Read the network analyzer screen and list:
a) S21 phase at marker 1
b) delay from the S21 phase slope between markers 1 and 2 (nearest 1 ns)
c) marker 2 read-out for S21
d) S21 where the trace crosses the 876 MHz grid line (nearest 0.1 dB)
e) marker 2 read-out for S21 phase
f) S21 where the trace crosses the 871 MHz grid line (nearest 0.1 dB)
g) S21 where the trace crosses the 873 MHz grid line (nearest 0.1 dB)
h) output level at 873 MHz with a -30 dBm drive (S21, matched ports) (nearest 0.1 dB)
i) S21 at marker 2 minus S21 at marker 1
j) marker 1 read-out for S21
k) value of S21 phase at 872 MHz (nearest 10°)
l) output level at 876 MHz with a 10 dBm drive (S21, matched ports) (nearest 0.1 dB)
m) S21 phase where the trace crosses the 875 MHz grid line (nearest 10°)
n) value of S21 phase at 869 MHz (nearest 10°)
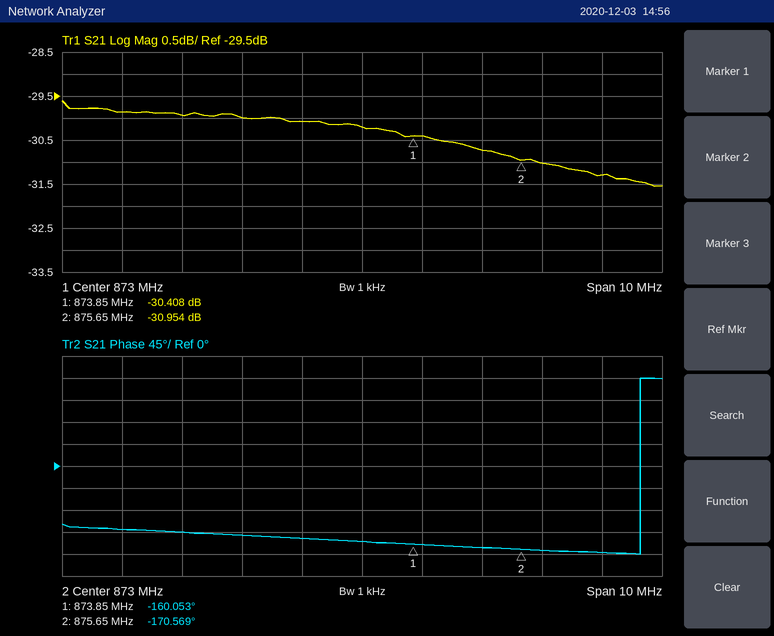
-160.053°
16 ns
-30.954 dB
-31.0 dB
-170.569°
-30.0 dB
-30.2 dB
-60.2 dBm
-0.546 dB
-30.408 dB
-150°
-21.0 dBm
-170°
-130°
